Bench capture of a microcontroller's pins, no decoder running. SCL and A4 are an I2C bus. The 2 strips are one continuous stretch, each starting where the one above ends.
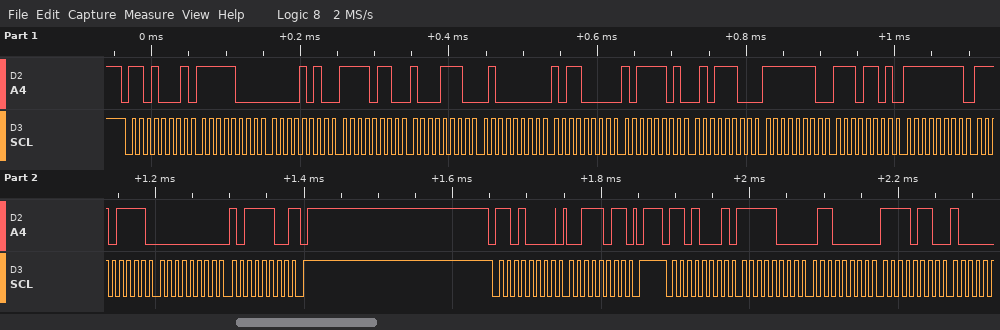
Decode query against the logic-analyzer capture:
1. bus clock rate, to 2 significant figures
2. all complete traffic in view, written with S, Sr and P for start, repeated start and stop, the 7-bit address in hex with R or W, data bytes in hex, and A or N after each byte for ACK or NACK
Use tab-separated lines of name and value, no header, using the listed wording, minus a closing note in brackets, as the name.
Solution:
bus clock rate, to 2 significant figures	100 kHz
all complete traffic in view, written with S, Sr and P for start, repeated start and stop, the 7-bit address in hex with R or W, data bytes in hex, and A or N after each byte for ACK or NACK	S 68R A F8 A 0A A F6 A 8E A 40 A B0 A BD A 5C A FE A ED A FF A EF A 00 A BC N P S 68W A 3B A P S 68R A F8 A 60 A F6 A
